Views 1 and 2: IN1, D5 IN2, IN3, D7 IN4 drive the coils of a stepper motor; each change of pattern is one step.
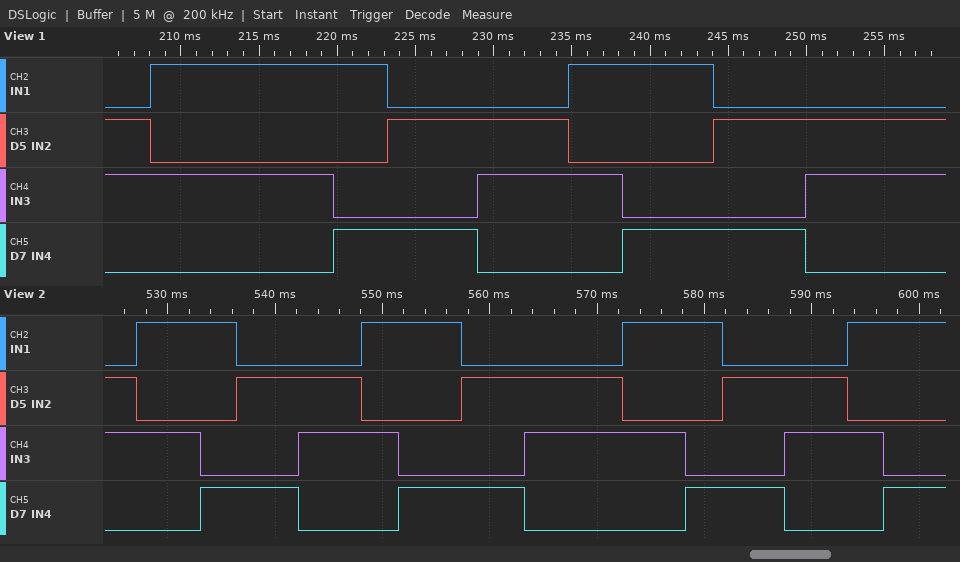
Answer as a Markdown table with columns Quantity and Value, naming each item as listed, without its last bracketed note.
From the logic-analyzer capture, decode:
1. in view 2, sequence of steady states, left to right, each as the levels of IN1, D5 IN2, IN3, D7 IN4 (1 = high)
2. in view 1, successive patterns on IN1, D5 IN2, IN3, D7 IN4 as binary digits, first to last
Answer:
| Quantity | Value |
|---|---|
| in view 2, sequence of steady states, left to right, each as the levels of IN1, D5 IN2, IN3, D7 IN4 | 0110 1010 1001 0101 0110 1010 1001 0101 0110 1010 1001 0101 0110 1010 1001 |
| in view 1, successive patterns on IN1, D5 IN2, IN3, D7 IN4 as binary digits, first to last | 0110 1010 1001 0101 0110 1010 1001 0101 0110 |
